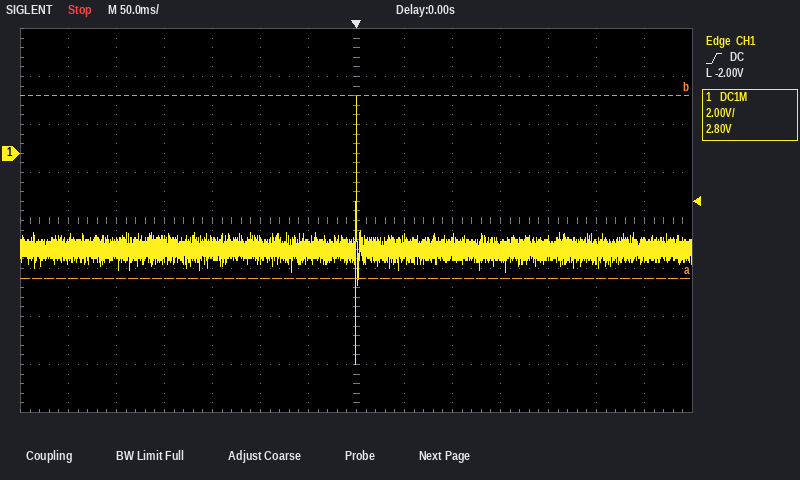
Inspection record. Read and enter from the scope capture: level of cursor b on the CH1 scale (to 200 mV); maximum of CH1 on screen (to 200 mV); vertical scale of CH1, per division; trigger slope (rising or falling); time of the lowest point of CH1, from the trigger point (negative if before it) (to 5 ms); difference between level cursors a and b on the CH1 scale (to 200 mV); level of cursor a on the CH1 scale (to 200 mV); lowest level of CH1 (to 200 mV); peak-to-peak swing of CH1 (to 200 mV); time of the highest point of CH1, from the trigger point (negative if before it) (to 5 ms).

2.4 V
2.4 V
2 V
rising
0 ms
7.6 V
-5.2 V
-8.8 V
11.2 V
0 ms
